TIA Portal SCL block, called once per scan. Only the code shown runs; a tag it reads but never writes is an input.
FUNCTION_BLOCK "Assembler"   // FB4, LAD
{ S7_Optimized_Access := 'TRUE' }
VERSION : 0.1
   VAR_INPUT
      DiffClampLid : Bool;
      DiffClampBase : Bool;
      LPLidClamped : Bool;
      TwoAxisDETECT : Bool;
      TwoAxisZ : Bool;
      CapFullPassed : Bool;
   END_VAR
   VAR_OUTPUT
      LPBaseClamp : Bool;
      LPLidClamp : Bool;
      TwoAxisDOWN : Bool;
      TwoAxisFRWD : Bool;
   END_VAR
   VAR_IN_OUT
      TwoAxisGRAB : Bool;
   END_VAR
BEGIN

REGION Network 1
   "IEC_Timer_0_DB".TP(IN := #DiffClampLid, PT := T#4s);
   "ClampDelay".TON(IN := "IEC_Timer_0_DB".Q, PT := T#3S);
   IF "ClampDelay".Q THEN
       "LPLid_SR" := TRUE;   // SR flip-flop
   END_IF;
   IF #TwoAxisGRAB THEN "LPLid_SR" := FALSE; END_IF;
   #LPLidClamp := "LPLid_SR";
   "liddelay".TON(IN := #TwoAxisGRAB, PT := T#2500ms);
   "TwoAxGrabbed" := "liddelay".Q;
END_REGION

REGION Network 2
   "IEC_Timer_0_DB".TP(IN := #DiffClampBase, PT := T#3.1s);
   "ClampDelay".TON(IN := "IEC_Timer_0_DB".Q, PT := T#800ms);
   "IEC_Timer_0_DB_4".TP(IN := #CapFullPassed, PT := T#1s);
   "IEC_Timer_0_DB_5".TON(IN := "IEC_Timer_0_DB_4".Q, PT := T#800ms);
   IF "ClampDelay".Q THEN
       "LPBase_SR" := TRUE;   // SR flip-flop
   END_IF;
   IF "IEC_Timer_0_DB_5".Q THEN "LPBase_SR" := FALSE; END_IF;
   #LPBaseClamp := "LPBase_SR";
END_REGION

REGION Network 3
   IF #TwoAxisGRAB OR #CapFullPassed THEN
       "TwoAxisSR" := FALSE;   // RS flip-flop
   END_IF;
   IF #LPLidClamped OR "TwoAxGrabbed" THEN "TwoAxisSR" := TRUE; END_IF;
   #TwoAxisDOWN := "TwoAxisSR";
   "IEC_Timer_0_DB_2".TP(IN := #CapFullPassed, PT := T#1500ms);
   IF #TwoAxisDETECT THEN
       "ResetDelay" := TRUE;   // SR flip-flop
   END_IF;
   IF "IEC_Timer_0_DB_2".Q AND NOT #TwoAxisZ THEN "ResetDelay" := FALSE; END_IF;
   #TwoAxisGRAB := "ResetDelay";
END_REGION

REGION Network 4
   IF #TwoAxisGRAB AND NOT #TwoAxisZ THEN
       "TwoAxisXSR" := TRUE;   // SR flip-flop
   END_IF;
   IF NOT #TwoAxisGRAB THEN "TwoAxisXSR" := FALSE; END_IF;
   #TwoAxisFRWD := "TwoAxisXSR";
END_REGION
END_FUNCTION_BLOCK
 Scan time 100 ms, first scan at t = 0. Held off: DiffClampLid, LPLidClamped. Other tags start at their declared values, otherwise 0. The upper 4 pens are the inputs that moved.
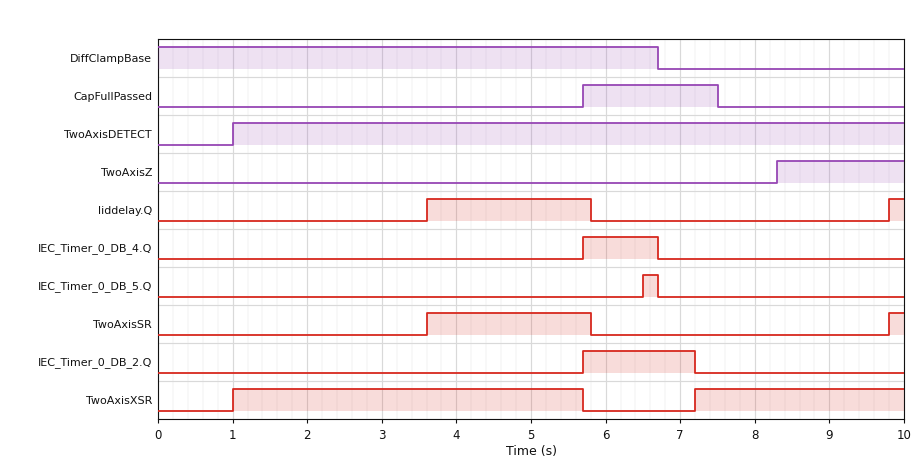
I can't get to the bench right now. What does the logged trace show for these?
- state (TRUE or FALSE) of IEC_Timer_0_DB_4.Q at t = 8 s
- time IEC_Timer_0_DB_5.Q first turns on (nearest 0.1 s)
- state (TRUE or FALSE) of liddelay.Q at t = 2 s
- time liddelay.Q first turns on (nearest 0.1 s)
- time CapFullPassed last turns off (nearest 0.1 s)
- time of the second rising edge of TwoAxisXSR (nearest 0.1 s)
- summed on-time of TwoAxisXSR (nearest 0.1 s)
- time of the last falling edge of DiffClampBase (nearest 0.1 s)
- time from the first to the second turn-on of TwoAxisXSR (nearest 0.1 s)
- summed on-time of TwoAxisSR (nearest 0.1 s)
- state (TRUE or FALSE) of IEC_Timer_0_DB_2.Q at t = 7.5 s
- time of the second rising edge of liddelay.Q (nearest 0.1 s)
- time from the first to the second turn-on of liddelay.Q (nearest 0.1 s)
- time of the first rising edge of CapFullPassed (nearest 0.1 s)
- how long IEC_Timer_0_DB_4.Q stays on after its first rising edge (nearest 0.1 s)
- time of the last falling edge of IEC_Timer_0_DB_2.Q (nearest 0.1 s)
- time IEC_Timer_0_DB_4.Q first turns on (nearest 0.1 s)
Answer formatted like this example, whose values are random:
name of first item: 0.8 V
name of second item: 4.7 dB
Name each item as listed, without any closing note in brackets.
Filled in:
state (TRUE or FALSE) of IEC_Timer_0_DB_4.Q at t = 8 s: FALSE
time IEC_Timer_0_DB_5.Q first turns on: 6.5 s
state (TRUE or FALSE) of liddelay.Q at t = 2 s: FALSE
time liddelay.Q first turns on: 3.6 s
time CapFullPassed last turns off: 7.5 s
time of the second rising edge of TwoAxisXSR: 7.2 s
summed on-time of TwoAxisXSR: 7.5 s
time of the last falling edge of DiffClampBase: 6.7 s
time from the first to the second turn-on of TwoAxisXSR: 6.2 s
summed on-time of TwoAxisSR: 2.4 s
state (TRUE or FALSE) of IEC_Timer_0_DB_2.Q at t = 7.5 s: FALSE
time of the second rising edge of liddelay.Q: 9.8 s
time from the first to the second turn-on of liddelay.Q: 6.2 s
time of the first rising edge of CapFullPassed: 5.7 s
how long IEC_Timer_0_DB_4.Q stays on after its first rising edge: 1.0 s
time of the last falling edge of IEC_Timer_0_DB_2.Q: 7.2 s
time IEC_Timer_0_DB_4.Q first turns on: 5.7 s
